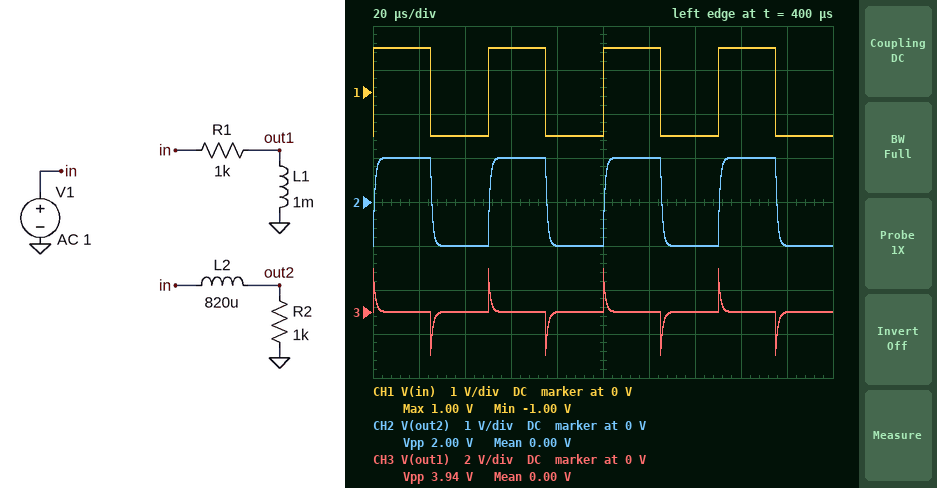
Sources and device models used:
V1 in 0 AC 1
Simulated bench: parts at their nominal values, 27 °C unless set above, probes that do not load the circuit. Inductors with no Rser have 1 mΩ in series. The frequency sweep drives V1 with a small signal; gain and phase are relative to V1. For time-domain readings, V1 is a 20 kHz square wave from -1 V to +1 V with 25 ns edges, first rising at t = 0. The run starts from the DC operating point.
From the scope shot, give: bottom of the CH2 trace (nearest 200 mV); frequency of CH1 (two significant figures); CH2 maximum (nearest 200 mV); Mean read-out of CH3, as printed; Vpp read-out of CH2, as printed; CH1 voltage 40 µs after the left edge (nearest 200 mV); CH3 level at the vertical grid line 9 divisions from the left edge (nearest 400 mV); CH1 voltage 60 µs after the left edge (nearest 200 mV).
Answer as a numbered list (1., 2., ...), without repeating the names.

1. -1.0 V
2. 20 kHz
3. 1.0 V
4. 0.00 V
5. 2.00 V
6. -1.0 V
7. 0 V
8. 1.0 V
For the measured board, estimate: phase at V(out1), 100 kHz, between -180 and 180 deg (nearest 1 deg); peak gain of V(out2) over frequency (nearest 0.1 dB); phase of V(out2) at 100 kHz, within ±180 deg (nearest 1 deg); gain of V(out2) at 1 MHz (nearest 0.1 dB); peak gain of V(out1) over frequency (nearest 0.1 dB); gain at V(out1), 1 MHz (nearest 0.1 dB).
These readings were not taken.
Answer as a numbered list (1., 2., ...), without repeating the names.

1. 58 deg
2. 0 dB
3. -27 deg
4. -14.4 dB
5. 0 dB
6. -0.1 dB
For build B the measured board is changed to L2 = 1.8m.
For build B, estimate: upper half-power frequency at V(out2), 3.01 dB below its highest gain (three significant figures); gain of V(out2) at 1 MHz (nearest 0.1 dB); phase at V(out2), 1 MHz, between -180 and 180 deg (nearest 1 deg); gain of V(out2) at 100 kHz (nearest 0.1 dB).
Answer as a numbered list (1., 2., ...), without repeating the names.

1. 88.4 kHz
2. -21.1 dB
3. -85 deg
4. -3.6 dB
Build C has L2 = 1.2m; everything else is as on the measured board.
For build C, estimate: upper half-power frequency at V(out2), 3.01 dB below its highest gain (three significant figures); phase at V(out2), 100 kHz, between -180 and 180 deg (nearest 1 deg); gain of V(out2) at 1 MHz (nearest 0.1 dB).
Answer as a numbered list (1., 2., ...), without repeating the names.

1. 133 kHz
2. -37 deg
3. -17.6 dB
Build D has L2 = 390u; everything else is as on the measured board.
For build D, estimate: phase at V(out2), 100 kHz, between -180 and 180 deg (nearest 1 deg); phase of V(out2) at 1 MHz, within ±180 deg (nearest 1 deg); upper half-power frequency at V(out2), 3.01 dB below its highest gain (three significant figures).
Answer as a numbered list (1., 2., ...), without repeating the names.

1. -14 deg
2. -68 deg
3. 408 kHz
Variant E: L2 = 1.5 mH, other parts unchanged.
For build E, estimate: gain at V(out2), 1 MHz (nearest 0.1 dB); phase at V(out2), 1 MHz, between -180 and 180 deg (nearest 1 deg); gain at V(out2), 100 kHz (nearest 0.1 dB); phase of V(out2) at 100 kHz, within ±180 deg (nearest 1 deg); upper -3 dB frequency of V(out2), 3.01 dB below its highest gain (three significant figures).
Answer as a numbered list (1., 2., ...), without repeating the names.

1. -19.5 dB
2. -84 deg
3. -2.8 dB
4. -43 deg
5. 106 kHz
